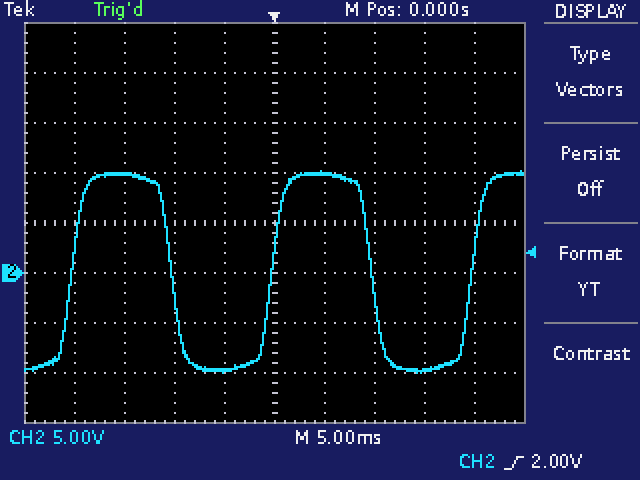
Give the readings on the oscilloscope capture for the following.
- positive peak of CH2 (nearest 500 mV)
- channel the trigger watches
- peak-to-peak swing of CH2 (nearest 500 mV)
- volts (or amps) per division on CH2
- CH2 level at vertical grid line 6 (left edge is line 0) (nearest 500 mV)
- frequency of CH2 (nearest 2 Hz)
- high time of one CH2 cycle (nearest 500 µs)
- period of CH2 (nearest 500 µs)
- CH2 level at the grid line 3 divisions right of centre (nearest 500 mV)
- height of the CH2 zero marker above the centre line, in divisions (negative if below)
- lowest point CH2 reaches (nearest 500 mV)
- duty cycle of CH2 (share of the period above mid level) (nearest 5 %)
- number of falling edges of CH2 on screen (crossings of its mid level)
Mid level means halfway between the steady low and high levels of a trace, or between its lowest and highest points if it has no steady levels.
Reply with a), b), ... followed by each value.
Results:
a) 10.0 V
b) CH2
c) 20.0 V
d) 5 V
e) 10.0 V
f) 50 Hz
g) 10.0 ms
h) 20.0 ms
i) -10.0 V
j) -1.0 div
k) -10.0 V
l) 50 %
m) 2
